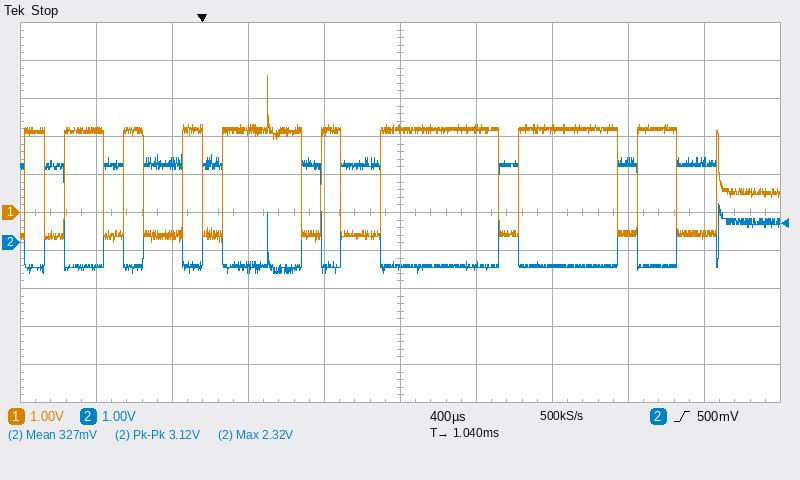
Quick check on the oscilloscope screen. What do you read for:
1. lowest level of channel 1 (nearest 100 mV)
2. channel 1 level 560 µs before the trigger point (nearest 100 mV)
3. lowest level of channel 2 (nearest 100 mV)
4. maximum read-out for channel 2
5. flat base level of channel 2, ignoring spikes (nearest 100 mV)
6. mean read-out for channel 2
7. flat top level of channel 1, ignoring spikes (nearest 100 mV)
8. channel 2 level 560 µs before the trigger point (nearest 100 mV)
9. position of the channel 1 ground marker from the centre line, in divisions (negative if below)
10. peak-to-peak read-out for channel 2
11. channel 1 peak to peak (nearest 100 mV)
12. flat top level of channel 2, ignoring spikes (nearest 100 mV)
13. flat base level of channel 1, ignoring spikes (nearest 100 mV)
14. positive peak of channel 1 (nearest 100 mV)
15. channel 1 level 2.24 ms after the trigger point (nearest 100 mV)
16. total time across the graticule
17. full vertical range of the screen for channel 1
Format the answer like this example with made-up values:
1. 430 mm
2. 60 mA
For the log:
1. -800 mV
2. 2.2 V
3. -800 mV
4. 2.32 V
5. -600 mV
6. 327 mV
7. 2.2 V
8. -600 mV
9. 0.0 div
10. 3.12 V
11. 4.4 V
12. 2.0 V
13. -600 mV
14. 3.6 V
15. -600 mV
16. 4 ms
17. 10 V
